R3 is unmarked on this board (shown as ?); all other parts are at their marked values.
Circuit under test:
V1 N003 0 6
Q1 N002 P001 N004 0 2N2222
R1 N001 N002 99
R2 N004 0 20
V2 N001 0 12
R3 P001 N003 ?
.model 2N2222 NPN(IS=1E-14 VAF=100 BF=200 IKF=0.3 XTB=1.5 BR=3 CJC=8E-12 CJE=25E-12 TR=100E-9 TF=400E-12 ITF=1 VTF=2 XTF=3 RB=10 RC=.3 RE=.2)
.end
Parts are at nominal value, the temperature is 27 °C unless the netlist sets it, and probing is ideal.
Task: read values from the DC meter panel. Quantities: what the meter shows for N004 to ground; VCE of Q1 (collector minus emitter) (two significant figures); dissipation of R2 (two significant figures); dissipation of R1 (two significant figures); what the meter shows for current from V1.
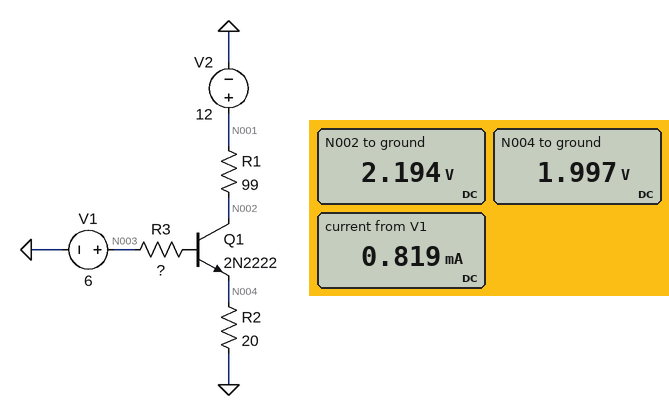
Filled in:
1.997 V
200 mV
200 mW
970 mW
0.819 mA
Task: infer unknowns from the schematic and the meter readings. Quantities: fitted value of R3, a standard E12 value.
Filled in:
3.9 kΩ
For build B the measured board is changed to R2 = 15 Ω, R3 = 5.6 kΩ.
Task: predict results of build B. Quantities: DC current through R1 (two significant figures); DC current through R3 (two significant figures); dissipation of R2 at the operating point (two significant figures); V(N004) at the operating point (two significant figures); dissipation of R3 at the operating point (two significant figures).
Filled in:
99 mA
660 µA
150 mW
1.5 V
2.4 mW
